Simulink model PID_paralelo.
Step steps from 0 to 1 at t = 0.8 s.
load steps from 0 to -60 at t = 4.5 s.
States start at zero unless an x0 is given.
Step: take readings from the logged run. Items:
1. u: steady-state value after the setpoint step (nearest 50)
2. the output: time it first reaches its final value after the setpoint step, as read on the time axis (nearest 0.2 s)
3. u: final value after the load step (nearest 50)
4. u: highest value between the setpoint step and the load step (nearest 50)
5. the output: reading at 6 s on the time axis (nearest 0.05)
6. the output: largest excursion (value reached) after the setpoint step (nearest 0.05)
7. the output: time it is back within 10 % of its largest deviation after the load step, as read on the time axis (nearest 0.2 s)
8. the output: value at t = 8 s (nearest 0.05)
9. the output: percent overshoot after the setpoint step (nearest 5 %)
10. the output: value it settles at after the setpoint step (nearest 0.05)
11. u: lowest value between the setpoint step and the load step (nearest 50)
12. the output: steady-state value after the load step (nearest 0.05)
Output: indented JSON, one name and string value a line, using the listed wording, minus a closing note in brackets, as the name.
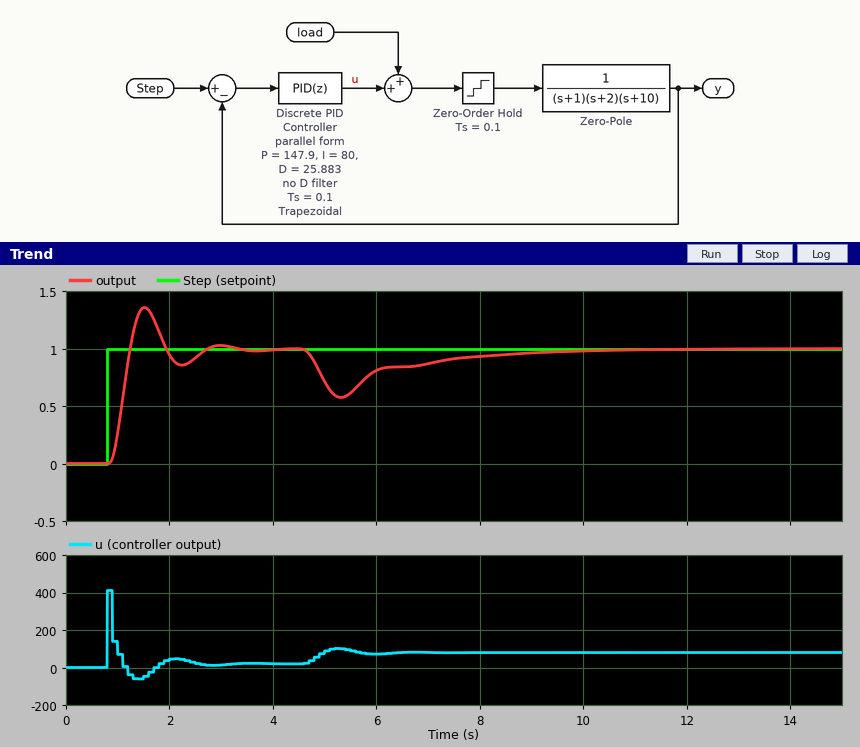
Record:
{
  "u: steady-state value after the setpoint step": "0",
  "the output: time it first reaches its final value after the setpoint step, as read on the time axis": "1.2 s",
  "u: final value after the load step": "100",
  "u: highest value between the setpoint step and the load step": "400",
  "the output: reading at 6 s on the time axis": "0.80",
  "the output: largest excursion (value reached) after the setpoint step": "1.35",
  "the output: time it is back within 10 % of its largest deviation after the load step, as read on the time axis": "8.8 s",
  "the output: value at t = 8 s": "0.95",
  "the output: percent overshoot after the setpoint step": "35 %",
  "the output: value it settles at after the setpoint step": "1.00",
  "u: lowest value between the setpoint step and the load step": "-50",
  "the output: steady-state value after the load step": "1.00"
}
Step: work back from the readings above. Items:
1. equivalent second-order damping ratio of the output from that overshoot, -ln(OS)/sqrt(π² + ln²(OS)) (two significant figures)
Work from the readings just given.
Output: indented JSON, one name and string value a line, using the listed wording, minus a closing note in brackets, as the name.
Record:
{
  "equivalent second-order damping ratio of the output from that overshoot, -ln(OS)/sqrt(π² + ln²(OS))": "0.32"
}
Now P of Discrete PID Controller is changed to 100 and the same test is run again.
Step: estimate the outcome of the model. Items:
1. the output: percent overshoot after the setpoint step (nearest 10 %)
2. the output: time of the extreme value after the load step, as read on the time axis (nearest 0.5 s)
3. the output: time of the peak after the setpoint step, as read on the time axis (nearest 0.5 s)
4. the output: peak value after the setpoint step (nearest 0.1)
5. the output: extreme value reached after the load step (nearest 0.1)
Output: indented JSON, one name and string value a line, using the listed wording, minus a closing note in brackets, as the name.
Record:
{
  "the output: percent overshoot after the setpoint step": "20 %",
  "the output: time of the extreme value after the load step, as read on the time axis": "5.5 s",
  "the output: time of the peak after the setpoint step, as read on the time axis": "1.5 s",
  "the output: peak value after the setpoint step": "1.2",
  "the output: extreme value reached after the load step": "0.5"
}
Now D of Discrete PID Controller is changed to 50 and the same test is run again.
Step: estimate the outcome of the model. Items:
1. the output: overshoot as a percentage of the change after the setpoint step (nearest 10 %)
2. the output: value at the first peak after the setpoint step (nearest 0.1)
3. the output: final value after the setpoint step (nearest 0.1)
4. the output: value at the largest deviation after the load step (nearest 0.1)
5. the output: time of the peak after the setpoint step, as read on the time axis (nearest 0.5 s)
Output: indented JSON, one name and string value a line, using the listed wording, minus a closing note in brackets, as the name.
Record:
{
  "the output: overshoot as a percentage of the change after the setpoint step": "30 %",
  "the output: value at the first peak after the setpoint step": "1.3",
  "the output: final value after the setpoint step": "1.0",
  "the output: value at the largest deviation after the load step": "0.7",
  "the output: time of the peak after the setpoint step, as read on the time axis": "1.5 s"
}
